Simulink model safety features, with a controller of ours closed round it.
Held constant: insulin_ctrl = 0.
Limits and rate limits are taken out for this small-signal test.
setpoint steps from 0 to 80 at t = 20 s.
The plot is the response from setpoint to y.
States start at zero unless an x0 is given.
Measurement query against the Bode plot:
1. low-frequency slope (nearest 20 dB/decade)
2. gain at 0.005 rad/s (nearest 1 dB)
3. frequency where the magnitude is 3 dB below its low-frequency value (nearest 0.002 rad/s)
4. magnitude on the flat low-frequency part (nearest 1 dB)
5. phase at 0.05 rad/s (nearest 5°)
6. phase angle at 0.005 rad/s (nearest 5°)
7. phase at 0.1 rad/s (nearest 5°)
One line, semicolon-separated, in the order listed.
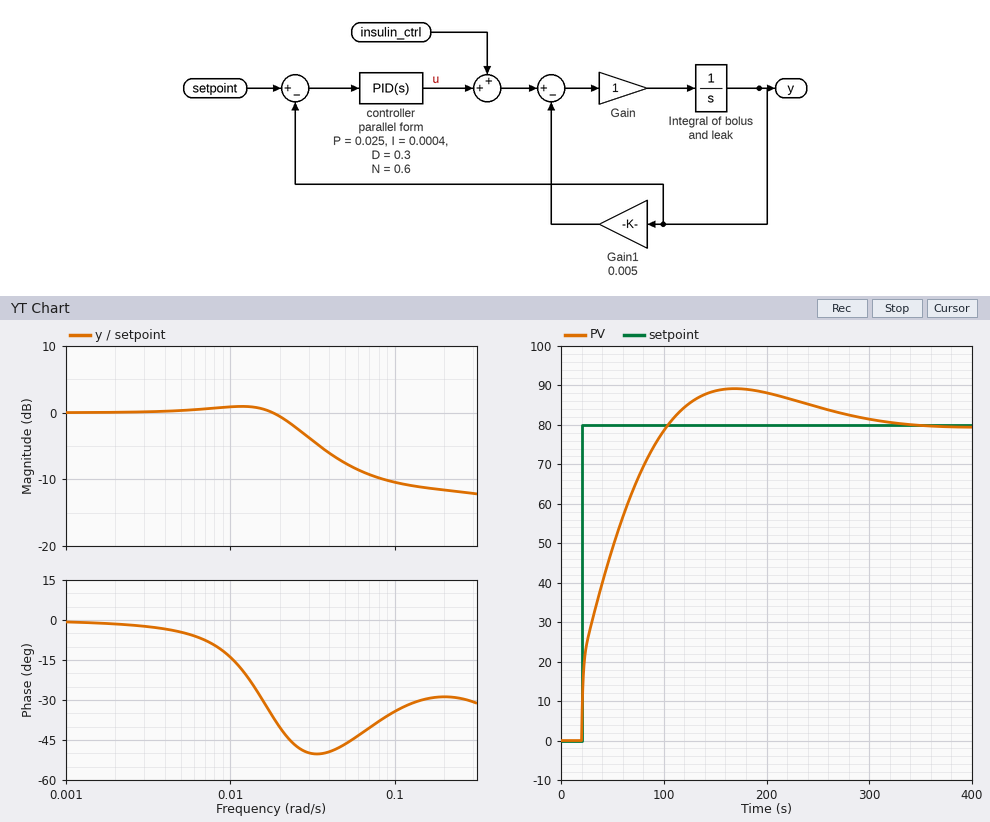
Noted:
0 dB/decade; 0 dB; 0.028 rad/s; 0 dB; -45°; -5°; -35°
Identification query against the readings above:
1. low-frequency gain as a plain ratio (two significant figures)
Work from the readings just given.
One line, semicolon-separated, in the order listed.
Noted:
1.0
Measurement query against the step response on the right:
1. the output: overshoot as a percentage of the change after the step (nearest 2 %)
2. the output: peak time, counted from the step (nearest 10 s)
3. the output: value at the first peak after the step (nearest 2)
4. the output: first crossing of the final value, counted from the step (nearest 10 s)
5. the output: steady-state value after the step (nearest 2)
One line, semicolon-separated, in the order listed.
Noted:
12 %; 150 s; 90; 80 s; 80
